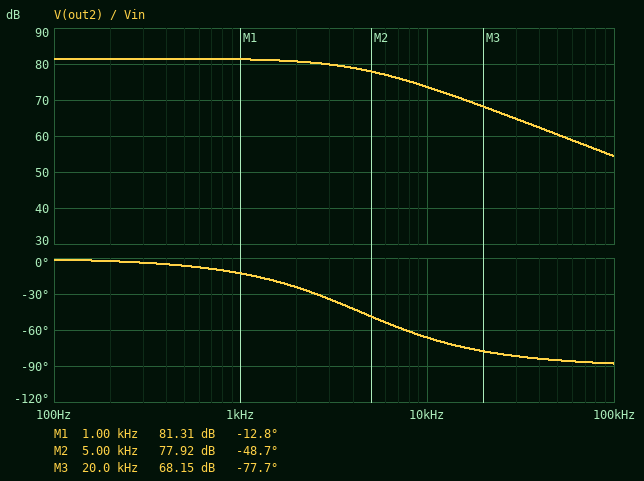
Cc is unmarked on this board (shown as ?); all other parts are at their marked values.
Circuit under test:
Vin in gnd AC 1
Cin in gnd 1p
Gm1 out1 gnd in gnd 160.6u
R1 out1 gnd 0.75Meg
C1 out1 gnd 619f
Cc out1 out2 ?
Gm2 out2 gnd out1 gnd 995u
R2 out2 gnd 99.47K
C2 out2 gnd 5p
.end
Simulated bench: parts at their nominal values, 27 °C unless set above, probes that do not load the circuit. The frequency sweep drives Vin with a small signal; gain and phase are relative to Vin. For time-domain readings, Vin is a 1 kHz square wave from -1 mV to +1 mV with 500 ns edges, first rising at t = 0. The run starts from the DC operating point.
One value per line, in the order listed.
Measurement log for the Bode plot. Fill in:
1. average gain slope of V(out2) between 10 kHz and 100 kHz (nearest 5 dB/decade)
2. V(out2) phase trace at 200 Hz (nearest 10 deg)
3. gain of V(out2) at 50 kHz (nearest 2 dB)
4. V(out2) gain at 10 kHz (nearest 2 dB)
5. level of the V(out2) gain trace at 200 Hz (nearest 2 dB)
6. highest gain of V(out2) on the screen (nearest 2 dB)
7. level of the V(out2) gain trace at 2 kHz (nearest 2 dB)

-20 dB/decade
0 deg
60 dB
74 dB
82 dB
82 dB
80 dB
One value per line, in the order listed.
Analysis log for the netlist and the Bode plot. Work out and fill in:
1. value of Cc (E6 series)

470 fF
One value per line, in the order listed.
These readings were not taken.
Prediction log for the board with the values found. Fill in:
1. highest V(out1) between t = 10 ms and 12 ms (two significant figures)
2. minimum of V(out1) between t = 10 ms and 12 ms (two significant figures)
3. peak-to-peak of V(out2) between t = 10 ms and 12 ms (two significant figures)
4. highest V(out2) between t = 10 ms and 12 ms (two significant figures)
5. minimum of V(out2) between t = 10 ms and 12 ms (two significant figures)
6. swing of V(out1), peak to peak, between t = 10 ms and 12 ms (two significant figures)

120 mV
-120 mV
24 V
12 V
-12 V
240 mV
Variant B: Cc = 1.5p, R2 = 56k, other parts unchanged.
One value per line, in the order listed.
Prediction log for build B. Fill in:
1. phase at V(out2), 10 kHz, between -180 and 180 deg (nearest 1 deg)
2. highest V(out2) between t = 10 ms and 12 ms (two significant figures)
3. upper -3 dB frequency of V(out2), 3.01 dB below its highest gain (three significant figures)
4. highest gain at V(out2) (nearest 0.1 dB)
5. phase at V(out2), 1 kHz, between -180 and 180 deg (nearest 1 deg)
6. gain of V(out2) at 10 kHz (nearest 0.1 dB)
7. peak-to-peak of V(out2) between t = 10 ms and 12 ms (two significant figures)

-76 deg
6.7 V
2.46 kHz
76.5 dB
-22 deg
64.1 dB
13 V
